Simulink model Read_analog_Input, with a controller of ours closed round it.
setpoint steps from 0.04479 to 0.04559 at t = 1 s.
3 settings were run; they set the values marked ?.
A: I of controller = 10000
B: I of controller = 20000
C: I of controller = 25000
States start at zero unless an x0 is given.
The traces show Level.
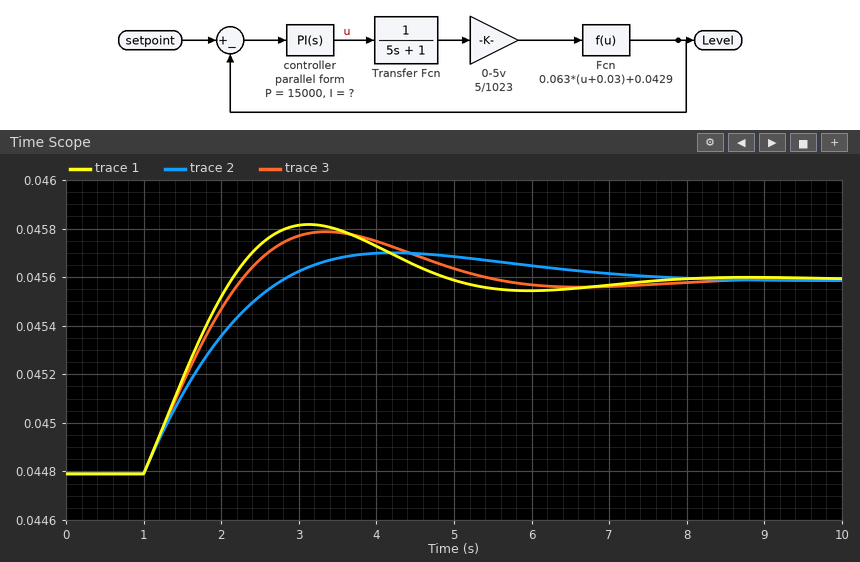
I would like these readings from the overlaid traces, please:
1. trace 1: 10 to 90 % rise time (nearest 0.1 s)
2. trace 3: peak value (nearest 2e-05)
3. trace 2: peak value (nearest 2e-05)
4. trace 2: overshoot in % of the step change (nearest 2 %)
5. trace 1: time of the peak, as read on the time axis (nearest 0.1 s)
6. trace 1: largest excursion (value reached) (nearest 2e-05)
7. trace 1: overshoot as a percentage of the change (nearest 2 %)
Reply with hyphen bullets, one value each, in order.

- 0.9 s
- 0.04578
- 0.04570
- 14 %
- 3.1 s
- 0.04582
- 28 %
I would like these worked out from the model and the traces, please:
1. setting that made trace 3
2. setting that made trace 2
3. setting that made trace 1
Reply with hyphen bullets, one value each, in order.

- B
- A
- C
